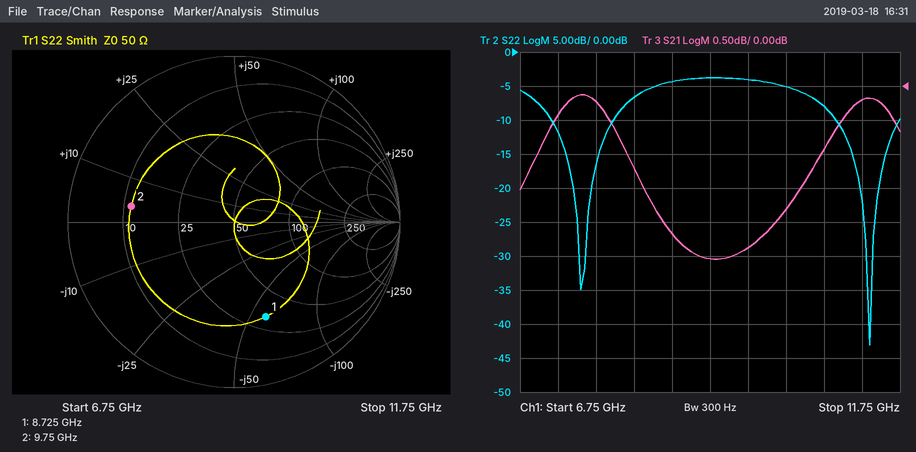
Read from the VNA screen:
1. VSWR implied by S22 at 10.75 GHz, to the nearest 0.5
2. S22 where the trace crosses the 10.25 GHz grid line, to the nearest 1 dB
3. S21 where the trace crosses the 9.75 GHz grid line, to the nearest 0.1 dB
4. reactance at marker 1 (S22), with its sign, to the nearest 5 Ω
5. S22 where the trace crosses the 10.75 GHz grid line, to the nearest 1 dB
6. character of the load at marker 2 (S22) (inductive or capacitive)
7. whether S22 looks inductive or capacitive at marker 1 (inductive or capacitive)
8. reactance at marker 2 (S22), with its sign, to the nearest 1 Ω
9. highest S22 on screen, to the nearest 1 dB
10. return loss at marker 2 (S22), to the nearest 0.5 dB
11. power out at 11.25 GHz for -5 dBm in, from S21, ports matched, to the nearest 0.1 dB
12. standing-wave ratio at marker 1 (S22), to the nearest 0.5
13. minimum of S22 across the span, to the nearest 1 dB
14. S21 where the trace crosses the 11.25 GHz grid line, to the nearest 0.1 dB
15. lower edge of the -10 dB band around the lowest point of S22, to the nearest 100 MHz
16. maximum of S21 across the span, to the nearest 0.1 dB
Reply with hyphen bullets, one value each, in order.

- 2.5
- -5 dB
- -2.4 dB
- -60 Ω
- -8 dB
- inductive
- capacitive
- +4 Ω
- -4 dB
- 4.0 dB
- -5.2 dBm
- 4.0
- -43 dB
- -0.2 dB
- 10.9 GHz
- -0.1 dB
